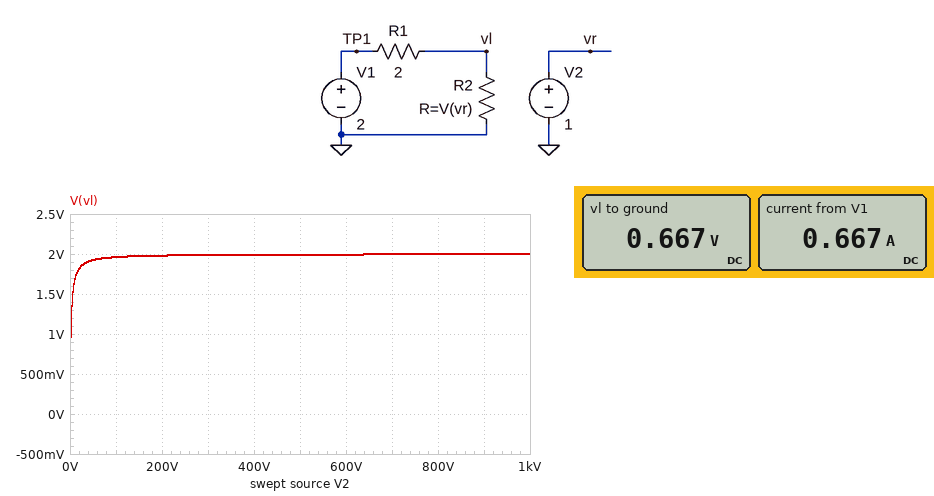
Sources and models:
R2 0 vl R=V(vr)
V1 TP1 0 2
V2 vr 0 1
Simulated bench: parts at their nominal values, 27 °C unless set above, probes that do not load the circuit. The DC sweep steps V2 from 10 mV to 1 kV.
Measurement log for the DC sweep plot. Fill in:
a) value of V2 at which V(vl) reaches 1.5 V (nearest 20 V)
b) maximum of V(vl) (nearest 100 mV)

0 V
2.0 V
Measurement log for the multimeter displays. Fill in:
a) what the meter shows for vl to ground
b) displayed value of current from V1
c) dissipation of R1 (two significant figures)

0.667 V
0.667 A
890 mW
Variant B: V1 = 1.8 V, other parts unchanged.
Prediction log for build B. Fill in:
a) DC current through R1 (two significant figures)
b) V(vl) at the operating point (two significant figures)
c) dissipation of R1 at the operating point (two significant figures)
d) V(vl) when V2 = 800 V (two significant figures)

600 mA
600 mV
720 mW
1.8 V
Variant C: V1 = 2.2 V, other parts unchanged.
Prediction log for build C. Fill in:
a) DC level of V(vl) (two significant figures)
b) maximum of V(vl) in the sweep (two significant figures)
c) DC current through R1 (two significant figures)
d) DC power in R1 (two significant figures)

730 mV
2.2 V
730 mA
1.1 W
